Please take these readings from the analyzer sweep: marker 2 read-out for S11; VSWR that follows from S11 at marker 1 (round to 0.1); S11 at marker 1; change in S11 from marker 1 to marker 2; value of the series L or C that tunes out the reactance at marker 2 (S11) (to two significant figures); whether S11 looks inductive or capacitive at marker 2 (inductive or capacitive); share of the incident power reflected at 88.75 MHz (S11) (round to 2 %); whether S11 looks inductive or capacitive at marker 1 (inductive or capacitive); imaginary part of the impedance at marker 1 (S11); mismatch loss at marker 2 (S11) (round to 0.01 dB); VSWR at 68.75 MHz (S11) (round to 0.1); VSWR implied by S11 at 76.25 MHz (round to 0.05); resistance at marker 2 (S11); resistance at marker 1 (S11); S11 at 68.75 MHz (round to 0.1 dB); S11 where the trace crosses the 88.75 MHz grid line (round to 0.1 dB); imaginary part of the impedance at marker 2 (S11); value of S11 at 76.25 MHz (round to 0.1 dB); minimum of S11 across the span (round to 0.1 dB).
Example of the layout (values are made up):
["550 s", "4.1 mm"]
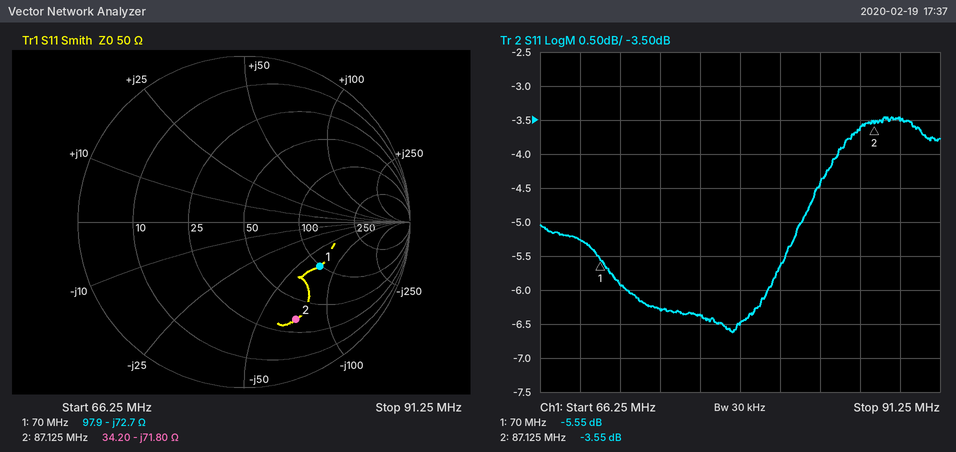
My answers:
["-3.55 dB", "3.2", "-5.55 dB", "2.00 dB", "130 nH", "capacitive", "44 %", "capacitive", "-72.7 Ω", "2.53 dB", "3.4", "2.85", "34.20 Ω", "97.9 Ω", "-5.3 dB", "-3.5 dB", "-71.80 Ω", "-6.4 dB", "-6.6 dB"]
